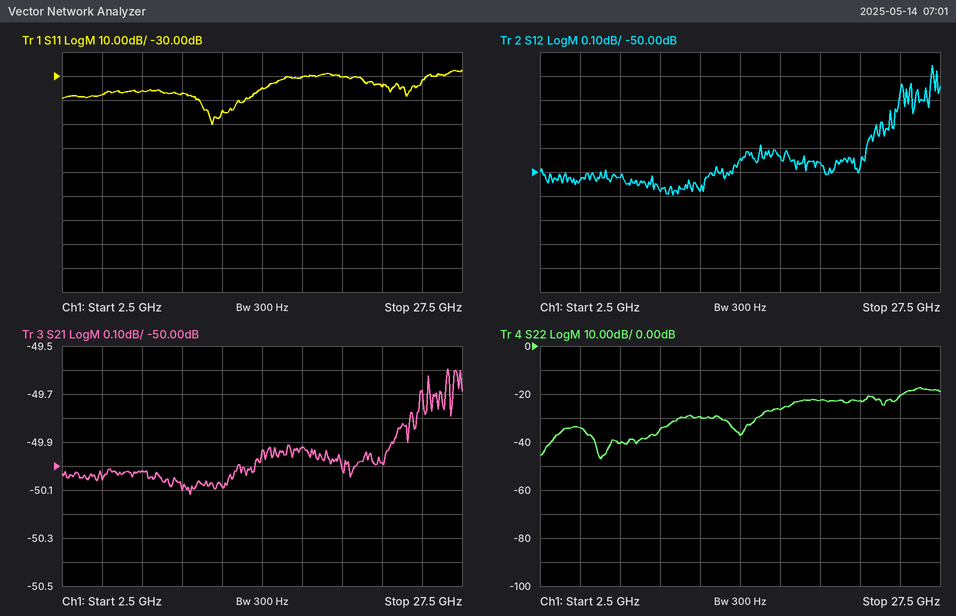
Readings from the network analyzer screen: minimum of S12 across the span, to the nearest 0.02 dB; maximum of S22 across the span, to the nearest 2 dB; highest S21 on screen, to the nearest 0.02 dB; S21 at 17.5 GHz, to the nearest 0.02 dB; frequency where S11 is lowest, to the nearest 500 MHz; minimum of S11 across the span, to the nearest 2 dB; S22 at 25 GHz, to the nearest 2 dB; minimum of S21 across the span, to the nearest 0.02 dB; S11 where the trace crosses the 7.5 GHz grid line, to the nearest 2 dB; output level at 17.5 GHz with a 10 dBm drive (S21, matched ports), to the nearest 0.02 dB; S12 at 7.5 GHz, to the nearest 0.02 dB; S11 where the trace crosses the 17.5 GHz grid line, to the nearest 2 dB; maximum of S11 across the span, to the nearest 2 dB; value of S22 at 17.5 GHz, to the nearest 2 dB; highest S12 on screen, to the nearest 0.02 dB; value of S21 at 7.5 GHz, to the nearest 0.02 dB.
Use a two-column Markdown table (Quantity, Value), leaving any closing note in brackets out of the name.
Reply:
| Quantity | Value |
|---|---|
| minimum of S12 across the span, to the nearest 0.02 dB | -50.10 dB |
| maximum of S22 across the span, to the nearest 2 dB | -18 dB |
| highest S21 on screen, to the nearest 0.02 dB | -49.60 dB |
| S21 at 17.5 GHz, to the nearest 0.02 dB | -49.92 dB |
| frequency where S11 is lowest, to the nearest 500 MHz | 12.0 GHz |
| minimum of S11 across the span, to the nearest 2 dB | -50 dB |
| S22 at 25 GHz, to the nearest 2 dB | -20 dB |
| minimum of S21 across the span, to the nearest 0.02 dB | -50.12 dB |
| S11 where the trace crosses the 7.5 GHz grid line, to the nearest 2 dB | -36 dB |
| output level at 17.5 GHz with a 10 dBm drive (S21, matched ports), to the nearest 0.02 dB | -39.92 dBm |
| S12 at 7.5 GHz, to the nearest 0.02 dB | -50.02 dB |
| S11 where the trace crosses the 17.5 GHz grid line, to the nearest 2 dB | -30 dB |
| maximum of S11 across the span, to the nearest 2 dB | -28 dB |
| value of S22 at 17.5 GHz, to the nearest 2 dB | -26 dB |
| highest S12 on screen, to the nearest 0.02 dB | -49.56 dB |
| value of S21 at 7.5 GHz, to the nearest 0.02 dB | -50.02 dB |
